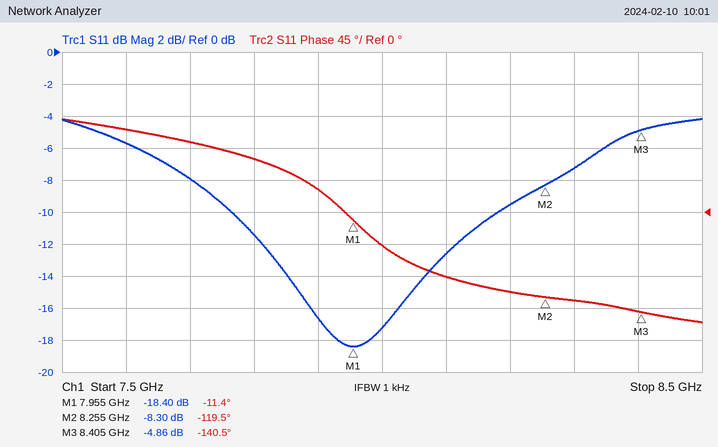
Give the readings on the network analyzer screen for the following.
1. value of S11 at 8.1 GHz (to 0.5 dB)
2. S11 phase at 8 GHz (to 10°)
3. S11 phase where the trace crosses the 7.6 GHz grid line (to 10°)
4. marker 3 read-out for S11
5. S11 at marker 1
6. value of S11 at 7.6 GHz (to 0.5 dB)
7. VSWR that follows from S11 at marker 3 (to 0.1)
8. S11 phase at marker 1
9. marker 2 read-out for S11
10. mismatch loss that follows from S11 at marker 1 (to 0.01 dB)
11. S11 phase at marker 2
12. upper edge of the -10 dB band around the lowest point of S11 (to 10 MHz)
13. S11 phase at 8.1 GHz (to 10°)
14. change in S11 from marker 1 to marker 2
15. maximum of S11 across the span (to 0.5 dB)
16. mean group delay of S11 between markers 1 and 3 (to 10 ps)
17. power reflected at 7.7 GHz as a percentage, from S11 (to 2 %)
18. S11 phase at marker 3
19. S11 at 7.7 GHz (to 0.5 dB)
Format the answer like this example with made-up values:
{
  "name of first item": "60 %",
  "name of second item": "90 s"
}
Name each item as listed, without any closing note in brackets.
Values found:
{
  "value of S11 at 8.1 GHz": "-12.5 dB",
  "S11 phase at 8 GHz": "-50°",
  "S11 phase where the trace crosses the 7.6 GHz grid line": "120°",
  "marker 3 read-out for S11": "-4.86 dB",
  "S11 at marker 1": "-18.40 dB",
  "value of S11 at 7.6 GHz": "-5.5 dB",
  "VSWR that follows from S11 at marker 3": "3.7",
  "S11 phase at marker 1": "-11.4°",
  "marker 2 read-out for S11": "-8.30 dB",
  "mismatch loss that follows from S11 at marker 1": "0.06 dB",
  "S11 phase at marker 2": "-119.5°",
  "upper edge of the -10 dB band around the lowest point of S11": "8.18 GHz",
  "S11 phase at 8.1 GHz": "-90°",
  "change in S11 from marker 1 to marker 2": "10.10 dB",
  "maximum of S11 across the span": "-4.0 dB",
  "mean group delay of S11 between markers 1 and 3": "800 ps",
  "power reflected at 7.7 GHz as a percentage, from S11": "16 %",
  "S11 phase at marker 3": "-140.5°",
  "S11 at 7.7 GHz": "-8.0 dB"
}
